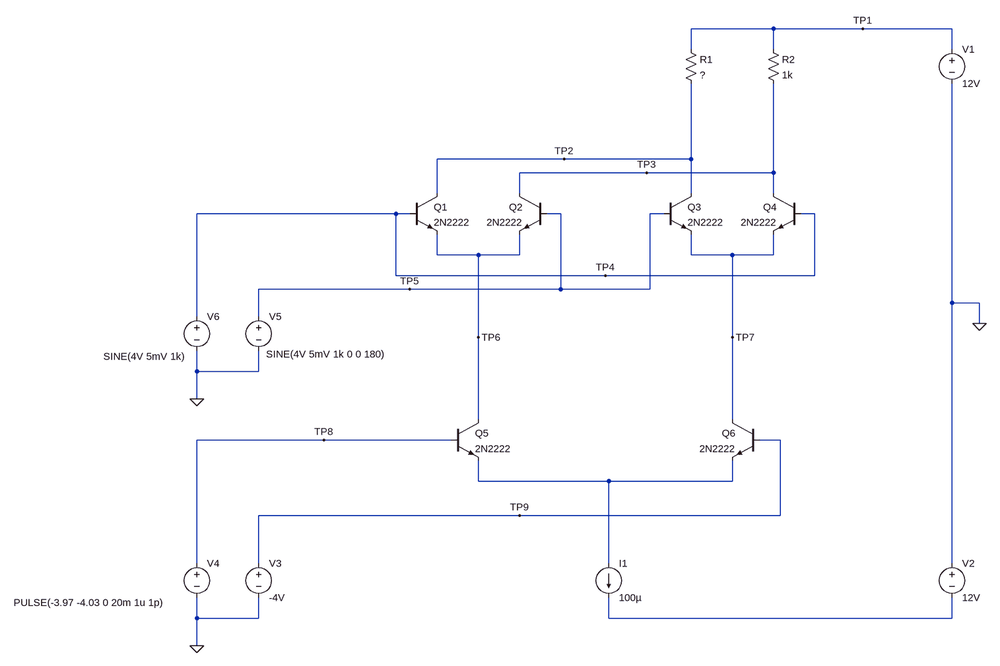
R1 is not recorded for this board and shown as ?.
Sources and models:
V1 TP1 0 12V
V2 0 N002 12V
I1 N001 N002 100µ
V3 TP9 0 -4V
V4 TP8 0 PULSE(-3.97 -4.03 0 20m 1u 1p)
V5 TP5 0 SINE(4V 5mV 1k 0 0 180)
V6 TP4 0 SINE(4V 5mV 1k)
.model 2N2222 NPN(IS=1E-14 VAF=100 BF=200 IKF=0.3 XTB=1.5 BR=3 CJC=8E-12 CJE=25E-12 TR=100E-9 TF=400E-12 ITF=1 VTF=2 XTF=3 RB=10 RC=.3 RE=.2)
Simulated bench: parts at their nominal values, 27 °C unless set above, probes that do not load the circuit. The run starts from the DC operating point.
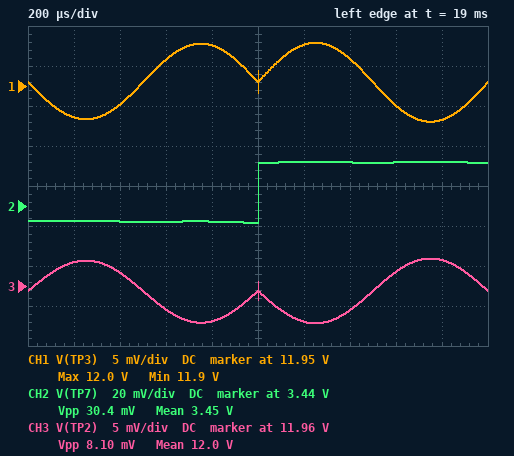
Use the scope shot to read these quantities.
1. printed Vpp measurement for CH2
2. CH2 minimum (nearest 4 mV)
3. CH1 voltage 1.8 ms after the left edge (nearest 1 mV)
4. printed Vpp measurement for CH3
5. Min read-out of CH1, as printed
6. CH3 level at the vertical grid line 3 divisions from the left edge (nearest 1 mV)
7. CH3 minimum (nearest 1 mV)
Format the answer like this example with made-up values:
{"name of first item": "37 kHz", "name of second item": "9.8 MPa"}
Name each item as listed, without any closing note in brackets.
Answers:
{"printed Vpp measurement for CH2": "30.4 mV", "CH2 minimum": "3.432 V", "CH1 voltage 1.8 ms after the left edge": "11.946 V", "printed Vpp measurement for CH3": "8.10 mV", "Min read-out of CH1, as printed": "11.9 V", "CH3 level at the vertical grid line 3 divisions from the left edge": "11.957 V", "CH3 minimum": "11.955 V"}
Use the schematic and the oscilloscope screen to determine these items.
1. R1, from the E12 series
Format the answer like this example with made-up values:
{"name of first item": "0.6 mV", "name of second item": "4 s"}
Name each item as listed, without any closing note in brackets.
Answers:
{"R1, from the E12 series": "820 Ω"}
